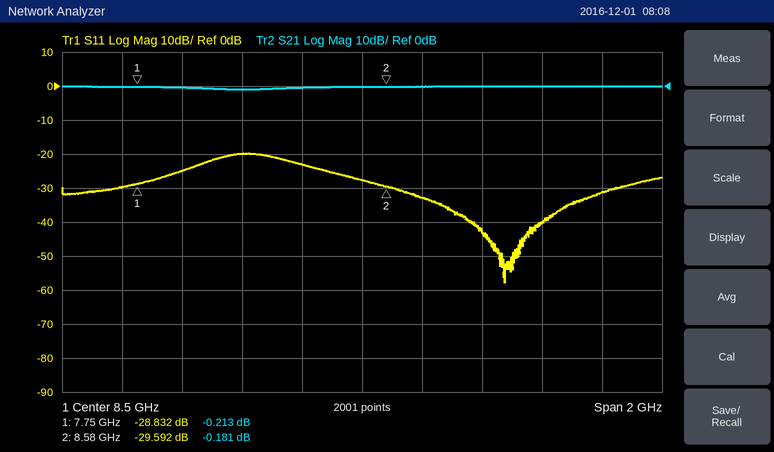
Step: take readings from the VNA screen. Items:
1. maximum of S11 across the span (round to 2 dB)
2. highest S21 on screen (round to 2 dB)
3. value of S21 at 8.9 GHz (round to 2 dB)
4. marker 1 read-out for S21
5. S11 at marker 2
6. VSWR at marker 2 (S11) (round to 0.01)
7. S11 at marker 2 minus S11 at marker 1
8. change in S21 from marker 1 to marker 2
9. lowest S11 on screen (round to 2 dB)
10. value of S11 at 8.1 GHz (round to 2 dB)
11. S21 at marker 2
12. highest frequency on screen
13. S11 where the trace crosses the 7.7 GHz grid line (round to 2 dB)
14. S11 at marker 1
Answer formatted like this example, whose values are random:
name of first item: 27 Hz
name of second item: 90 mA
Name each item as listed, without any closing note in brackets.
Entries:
maximum of S11 across the span: -20 dB
highest S21 on screen: 0 dB
value of S21 at 8.9 GHz: 0 dB
marker 1 read-out for S21: -0.213 dB
S11 at marker 2: -29.592 dB
VSWR at marker 2 (S11): 1.07
S11 at marker 2 minus S11 at marker 1: -0.760 dB
change in S21 from marker 1 to marker 2: 0.032 dB
lowest S11 on screen: -58 dB
value of S11 at 8.1 GHz: -20 dB
S21 at marker 2: -0.181 dB
highest frequency on screen: 9.5 GHz
S11 where the trace crosses the 7.7 GHz grid line: -30 dB
S11 at marker 1: -28.832 dB
